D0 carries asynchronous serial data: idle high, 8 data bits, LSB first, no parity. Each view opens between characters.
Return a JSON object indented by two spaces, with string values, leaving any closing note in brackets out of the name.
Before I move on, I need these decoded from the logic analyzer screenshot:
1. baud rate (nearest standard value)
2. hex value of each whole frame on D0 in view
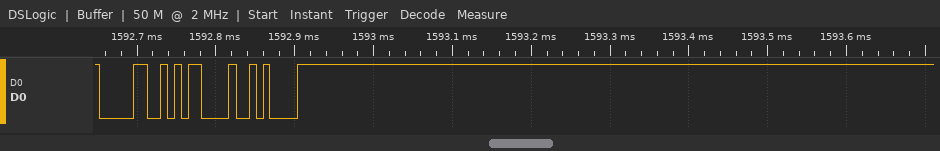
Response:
{
  "baud rate": "115200 baud",
  "hex value of each whole frame on D0 in view": "30, 0D, 0A"
}
